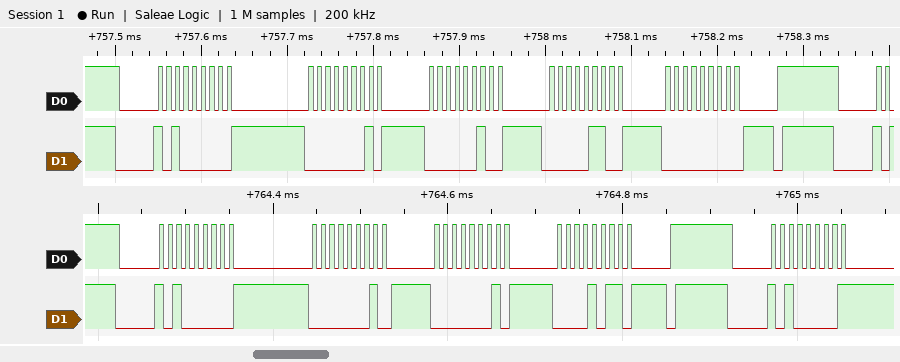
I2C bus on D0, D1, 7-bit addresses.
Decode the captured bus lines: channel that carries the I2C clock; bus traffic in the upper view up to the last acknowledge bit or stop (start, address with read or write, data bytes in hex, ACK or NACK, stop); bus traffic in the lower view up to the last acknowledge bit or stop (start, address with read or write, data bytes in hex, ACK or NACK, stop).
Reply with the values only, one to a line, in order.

D0
start, address 50 write ACK, 01 ACK, 02 ACK, 06 ACK, 00 ACK, stop
start, address 50 write ACK, 01 ACK, 01 ACK, 0B ACK, stop, start, address 50 write NACK
